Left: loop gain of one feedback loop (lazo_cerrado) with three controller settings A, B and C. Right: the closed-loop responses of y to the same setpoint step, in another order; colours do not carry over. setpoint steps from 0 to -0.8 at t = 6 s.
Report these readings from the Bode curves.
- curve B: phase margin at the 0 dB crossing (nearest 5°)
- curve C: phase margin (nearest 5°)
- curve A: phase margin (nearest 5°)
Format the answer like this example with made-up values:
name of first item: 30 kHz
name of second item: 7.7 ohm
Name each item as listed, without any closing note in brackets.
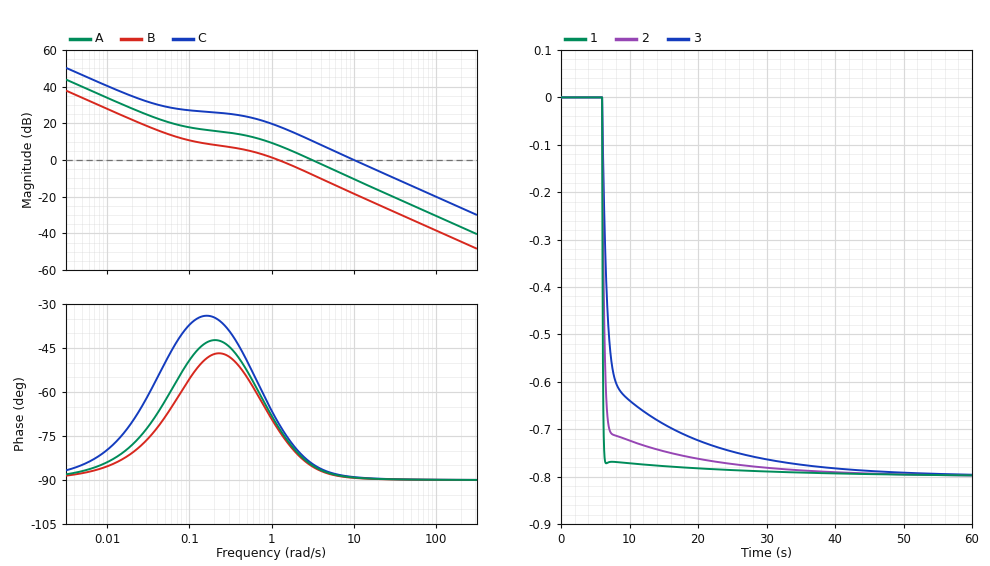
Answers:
curve B: phase margin at the 0 dB crossing: 105°
curve C: phase margin: 90°
curve A: phase margin: 95°
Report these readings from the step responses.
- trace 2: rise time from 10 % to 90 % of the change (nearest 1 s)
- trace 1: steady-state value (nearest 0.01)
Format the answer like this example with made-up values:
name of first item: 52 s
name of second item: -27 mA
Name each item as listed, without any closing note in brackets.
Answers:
trace 2: rise time from 10 % to 90 % of the change: 3 s
trace 1: steady-state value: -0.80
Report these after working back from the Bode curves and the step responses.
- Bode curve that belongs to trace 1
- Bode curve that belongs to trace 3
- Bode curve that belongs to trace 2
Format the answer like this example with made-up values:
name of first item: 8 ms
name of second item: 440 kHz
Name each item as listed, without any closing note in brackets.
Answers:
Bode curve that belongs to trace 1: C
Bode curve that belongs to trace 3: B
Bode curve that belongs to trace 2: A
